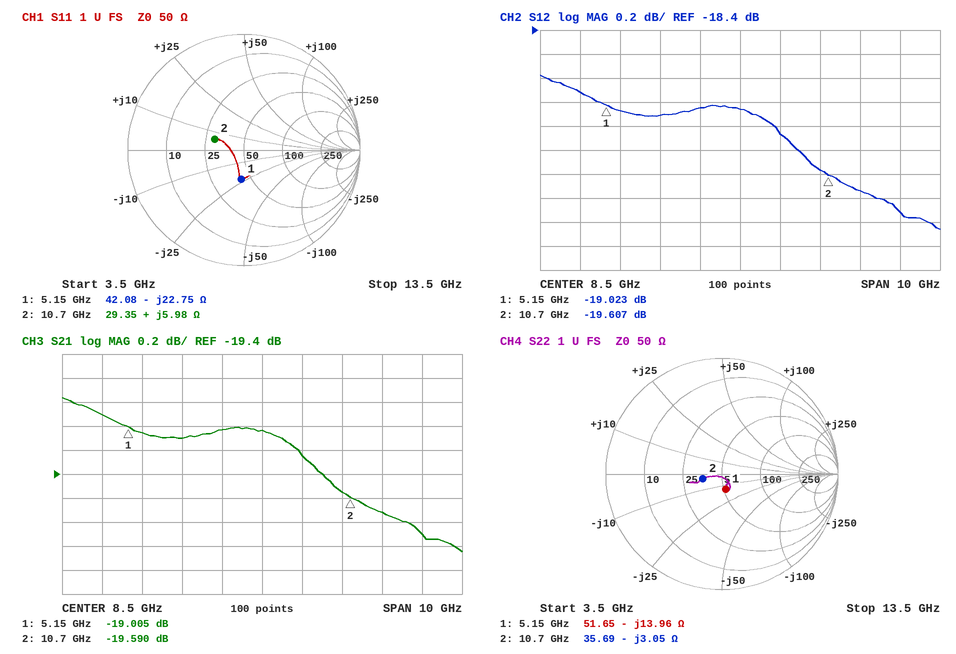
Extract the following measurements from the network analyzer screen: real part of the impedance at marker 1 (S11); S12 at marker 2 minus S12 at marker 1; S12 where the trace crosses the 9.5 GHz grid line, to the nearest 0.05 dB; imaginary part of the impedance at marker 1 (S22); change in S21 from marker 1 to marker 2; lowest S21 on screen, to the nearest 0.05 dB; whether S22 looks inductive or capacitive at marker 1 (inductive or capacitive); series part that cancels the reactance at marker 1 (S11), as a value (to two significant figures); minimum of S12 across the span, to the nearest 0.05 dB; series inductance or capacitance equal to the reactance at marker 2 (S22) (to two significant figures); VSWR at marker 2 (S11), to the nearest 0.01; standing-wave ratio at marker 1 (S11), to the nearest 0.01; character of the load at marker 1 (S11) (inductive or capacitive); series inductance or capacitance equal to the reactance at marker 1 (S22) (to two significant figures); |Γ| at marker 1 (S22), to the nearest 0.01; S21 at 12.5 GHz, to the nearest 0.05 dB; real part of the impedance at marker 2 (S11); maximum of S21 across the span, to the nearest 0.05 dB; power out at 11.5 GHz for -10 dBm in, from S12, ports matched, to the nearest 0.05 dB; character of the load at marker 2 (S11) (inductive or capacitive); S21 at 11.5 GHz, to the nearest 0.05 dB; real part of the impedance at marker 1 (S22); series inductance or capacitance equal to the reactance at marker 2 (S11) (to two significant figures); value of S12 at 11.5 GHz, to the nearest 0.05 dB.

42.08 Ω
-0.584 dB
-19.25 dB
-13.96 Ω
-0.585 dB
-20.05 dB
capacitive
700 pH
-20.05 dB
4.9 pF
1.74
1.68
capacitive
2.2 pF
0.14
-19.90 dB
29.35 Ω
-18.75 dB
-29.75 dBm
inductive
-19.70 dB
51.65 Ω
89 pH
-19.75 dB
